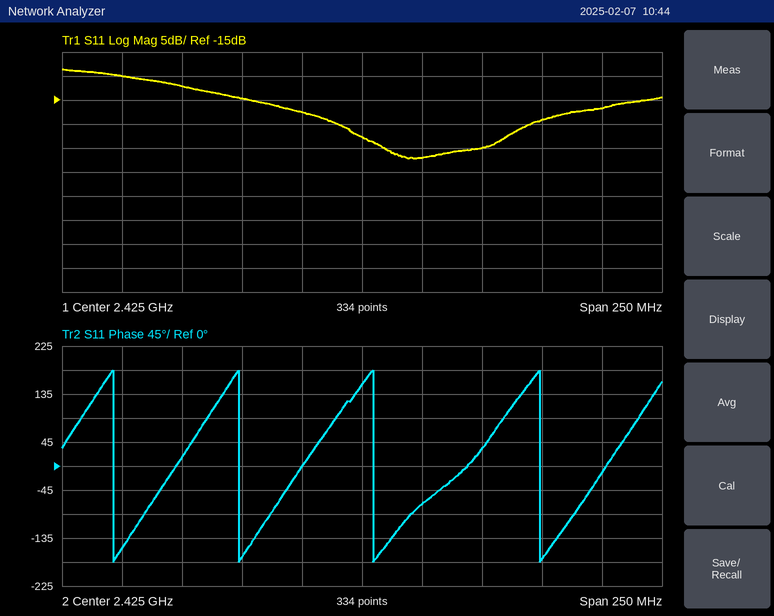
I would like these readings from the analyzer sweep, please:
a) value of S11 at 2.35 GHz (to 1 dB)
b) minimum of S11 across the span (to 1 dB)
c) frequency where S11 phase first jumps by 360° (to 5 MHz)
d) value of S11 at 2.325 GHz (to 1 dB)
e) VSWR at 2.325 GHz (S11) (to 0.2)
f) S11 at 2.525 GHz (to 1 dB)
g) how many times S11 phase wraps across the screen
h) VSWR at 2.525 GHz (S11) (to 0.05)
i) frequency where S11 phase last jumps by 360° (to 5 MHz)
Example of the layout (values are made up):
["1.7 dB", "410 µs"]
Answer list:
["-12 dB", "-27 dB", "2.320 GHz", "-10 dB", "2.0", "-17 dB", "4", "1.35", "2.500 GHz"]
